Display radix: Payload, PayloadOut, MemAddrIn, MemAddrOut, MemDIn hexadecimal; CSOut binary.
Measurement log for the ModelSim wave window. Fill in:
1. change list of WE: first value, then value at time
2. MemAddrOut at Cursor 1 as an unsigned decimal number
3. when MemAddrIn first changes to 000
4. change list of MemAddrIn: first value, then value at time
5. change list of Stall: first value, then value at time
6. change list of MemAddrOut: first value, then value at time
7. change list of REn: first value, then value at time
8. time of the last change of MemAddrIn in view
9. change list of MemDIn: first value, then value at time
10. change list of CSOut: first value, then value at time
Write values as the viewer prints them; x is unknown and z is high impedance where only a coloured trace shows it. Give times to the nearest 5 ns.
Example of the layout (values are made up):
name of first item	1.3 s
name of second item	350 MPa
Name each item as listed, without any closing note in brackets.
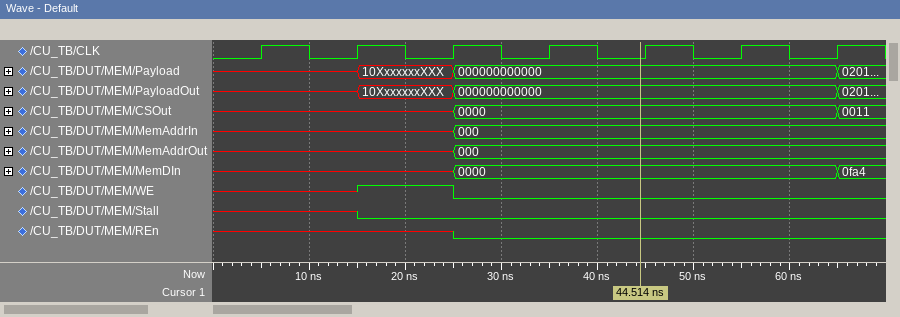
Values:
change list of WE: first value, then value at time	x, 1 at 15 ns, 0 at 25 ns
MemAddrOut at Cursor 1 as an unsigned decimal number	0
when MemAddrIn first changes to 000	25 ns
change list of MemAddrIn: first value, then value at time	x, 000 at 25 ns
change list of Stall: first value, then value at time	x, 0 at 15 ns
change list of MemAddrOut: first value, then value at time	x, 000 at 25 ns
change list of REn: first value, then value at time	x, 0 at 25 ns
time of the last change of MemAddrIn in view	25 ns
change list of MemDIn: first value, then value at time	x, 0000 at 25 ns, 0fa4 at 65 ns
change list of CSOut: first value, then value at time	x, 0000 at 25 ns, 0011 at 65 ns
